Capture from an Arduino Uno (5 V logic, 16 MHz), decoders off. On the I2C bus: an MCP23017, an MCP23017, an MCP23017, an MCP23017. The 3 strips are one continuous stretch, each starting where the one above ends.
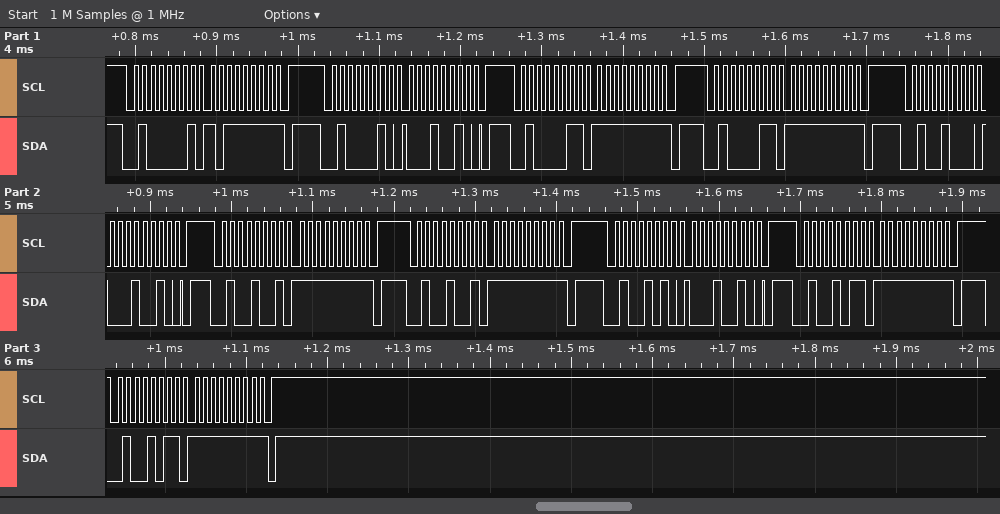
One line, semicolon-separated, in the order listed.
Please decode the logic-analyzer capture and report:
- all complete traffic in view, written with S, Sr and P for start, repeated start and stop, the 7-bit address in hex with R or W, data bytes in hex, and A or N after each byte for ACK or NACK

S 20R A BF N P S 21W A 12 A P S 21R A FF N P S 21R A FF N P S 24W A 12 A P S 24R A FF N P S 24R A FF N P S 25W A 12 A P S 25R A FF N P S 25R A FF N P
